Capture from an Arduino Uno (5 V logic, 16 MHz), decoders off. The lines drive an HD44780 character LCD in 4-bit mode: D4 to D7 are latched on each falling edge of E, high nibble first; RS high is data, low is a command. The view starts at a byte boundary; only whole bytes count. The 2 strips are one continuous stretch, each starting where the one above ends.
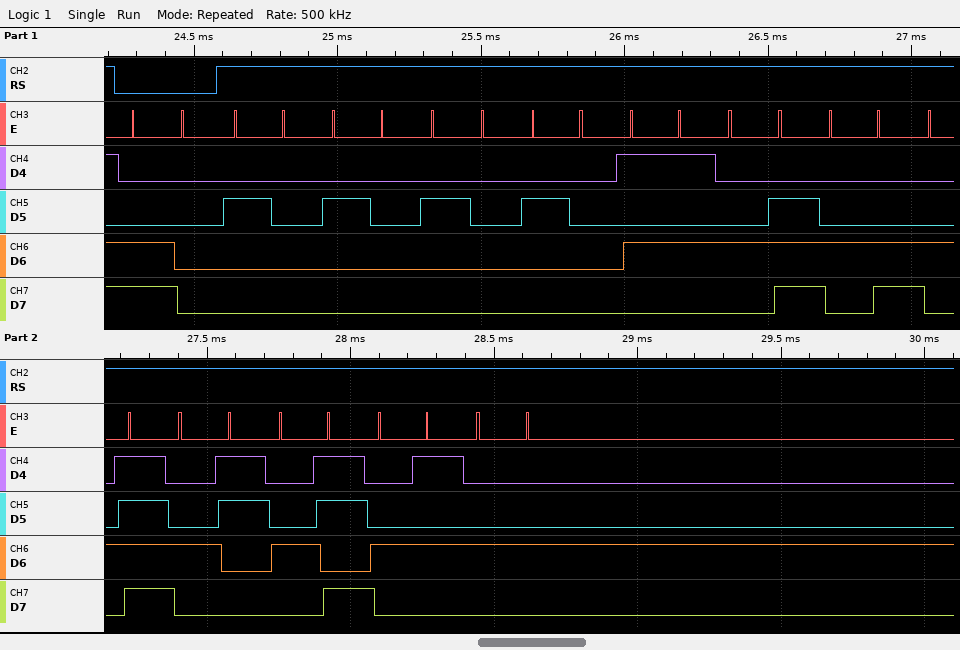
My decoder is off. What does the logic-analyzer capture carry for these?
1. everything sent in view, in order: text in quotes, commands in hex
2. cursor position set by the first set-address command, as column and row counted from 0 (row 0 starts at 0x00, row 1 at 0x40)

0xC0 "    UNLOCKED"
column 0, row 1
